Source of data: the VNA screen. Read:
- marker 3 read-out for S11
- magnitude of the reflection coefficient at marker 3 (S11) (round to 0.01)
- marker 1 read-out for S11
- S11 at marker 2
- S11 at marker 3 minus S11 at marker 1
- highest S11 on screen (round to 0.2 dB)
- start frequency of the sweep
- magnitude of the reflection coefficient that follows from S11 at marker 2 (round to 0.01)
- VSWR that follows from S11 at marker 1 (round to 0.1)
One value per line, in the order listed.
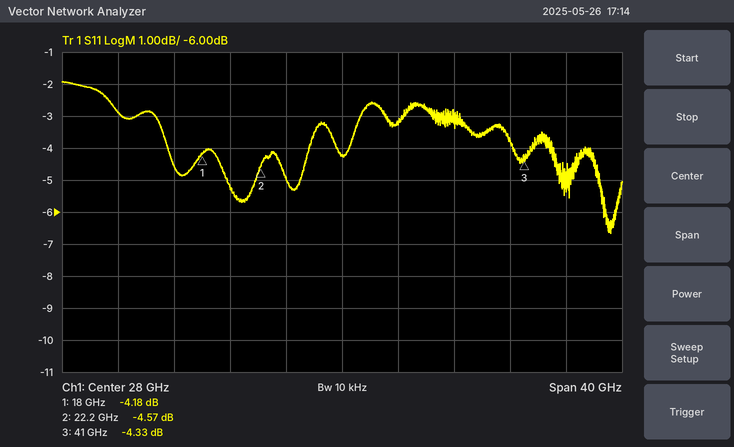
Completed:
-4.33 dB
0.61
-4.18 dB
-4.57 dB
-0.15 dB
-2.0 dB
8 GHz
0.59
4.2
